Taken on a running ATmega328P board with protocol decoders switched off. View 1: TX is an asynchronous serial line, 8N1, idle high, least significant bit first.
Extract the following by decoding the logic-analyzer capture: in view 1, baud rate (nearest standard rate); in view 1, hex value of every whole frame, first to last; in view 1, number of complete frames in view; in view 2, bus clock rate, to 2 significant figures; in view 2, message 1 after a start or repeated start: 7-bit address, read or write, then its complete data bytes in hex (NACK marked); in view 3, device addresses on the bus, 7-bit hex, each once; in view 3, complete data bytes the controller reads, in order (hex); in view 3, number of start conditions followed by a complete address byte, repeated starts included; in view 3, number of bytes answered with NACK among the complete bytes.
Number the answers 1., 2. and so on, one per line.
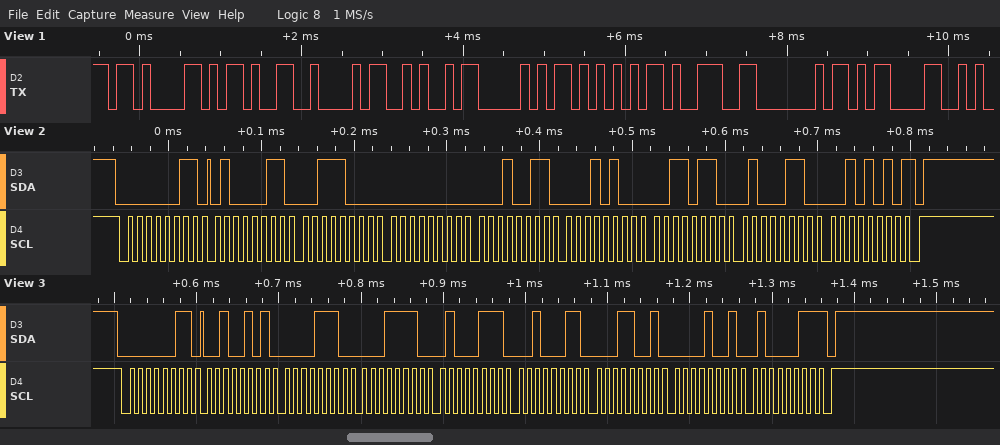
1. 9600 baud
2. 0B 2D 42 4A 50 55 39 40 0D
3. 9
4. 100 kHz
5. 0x01 read: 43 38 00 13 14 36 46 2A NACK
6. 0x01
7. 25 0E 1E 47 23 19 09 43
8. 1
9. 1
